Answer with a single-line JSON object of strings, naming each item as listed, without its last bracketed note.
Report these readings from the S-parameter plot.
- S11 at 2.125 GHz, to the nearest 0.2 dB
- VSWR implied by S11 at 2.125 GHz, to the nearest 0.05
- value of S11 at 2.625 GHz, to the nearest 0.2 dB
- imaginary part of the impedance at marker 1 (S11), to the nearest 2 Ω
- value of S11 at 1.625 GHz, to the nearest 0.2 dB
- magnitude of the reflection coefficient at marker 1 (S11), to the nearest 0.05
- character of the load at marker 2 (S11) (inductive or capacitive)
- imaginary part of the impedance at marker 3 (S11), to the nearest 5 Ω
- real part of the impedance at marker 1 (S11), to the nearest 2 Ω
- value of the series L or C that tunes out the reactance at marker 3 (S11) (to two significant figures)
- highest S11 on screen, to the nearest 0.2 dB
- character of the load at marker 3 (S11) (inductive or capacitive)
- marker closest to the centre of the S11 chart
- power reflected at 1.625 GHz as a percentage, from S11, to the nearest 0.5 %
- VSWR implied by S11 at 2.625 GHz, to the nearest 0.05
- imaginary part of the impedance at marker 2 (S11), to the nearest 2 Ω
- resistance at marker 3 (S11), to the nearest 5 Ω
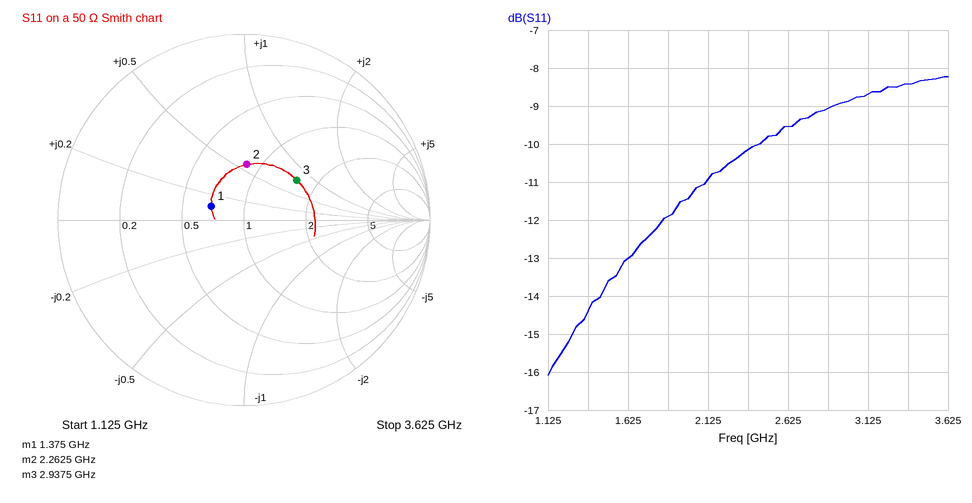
{"S11 at 2.125 GHz, to the nearest 0.2 dB": "-11.0 dB", "VSWR implied by S11 at 2.125 GHz, to the nearest 0.05": "1.80", "value of S11 at 2.625 GHz, to the nearest 0.2 dB": "-9.6 dB", "imaginary part of the impedance at marker 1 (S11), to the nearest 2 Ω": "+6 Ω", "value of S11 at 1.625 GHz, to the nearest 0.2 dB": "-13.0 dB", "magnitude of the reflection coefficient at marker 1 (S11), to the nearest 0.05": "0.20", "character of the load at marker 2 (S11)": "inductive", "imaginary part of the impedance at marker 3 (S11), to the nearest 5 Ω": "+40 Ω", "real part of the impedance at marker 1 (S11), to the nearest 2 Ω": "34 Ω", "value of the series L or C that tunes out the reactance at marker 3 (S11)": "1.4 pF", "highest S11 on screen, to the nearest 0.2 dB": "-8.2 dB", "character of the load at marker 3 (S11)": "inductive", "marker closest to the centre of the S11 chart": "marker 1", "power reflected at 1.625 GHz as a percentage, from S11, to the nearest 0.5 %": "5.0 %", "VSWR implied by S11 at 2.625 GHz, to the nearest 0.05": "2.00", "imaginary part of the impedance at marker 2 (S11), to the nearest 2 Ω": "+28 Ω", "resistance at marker 3 (S11), to the nearest 5 Ω": "80 Ω"}
